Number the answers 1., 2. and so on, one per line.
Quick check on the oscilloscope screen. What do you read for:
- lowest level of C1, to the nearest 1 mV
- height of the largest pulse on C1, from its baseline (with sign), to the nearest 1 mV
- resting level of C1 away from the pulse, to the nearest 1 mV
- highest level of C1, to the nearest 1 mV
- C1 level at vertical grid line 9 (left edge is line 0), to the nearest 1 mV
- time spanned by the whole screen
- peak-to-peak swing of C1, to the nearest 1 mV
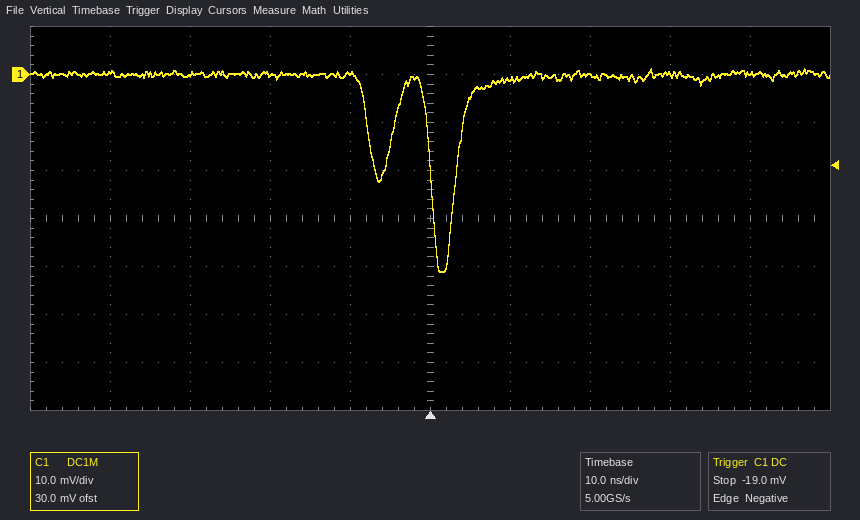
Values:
1. -41 mV
2. -41 mV
3. 0 mV
4. 1 mV
5. 0 mV
6. 100 ns
7. 42 mV
